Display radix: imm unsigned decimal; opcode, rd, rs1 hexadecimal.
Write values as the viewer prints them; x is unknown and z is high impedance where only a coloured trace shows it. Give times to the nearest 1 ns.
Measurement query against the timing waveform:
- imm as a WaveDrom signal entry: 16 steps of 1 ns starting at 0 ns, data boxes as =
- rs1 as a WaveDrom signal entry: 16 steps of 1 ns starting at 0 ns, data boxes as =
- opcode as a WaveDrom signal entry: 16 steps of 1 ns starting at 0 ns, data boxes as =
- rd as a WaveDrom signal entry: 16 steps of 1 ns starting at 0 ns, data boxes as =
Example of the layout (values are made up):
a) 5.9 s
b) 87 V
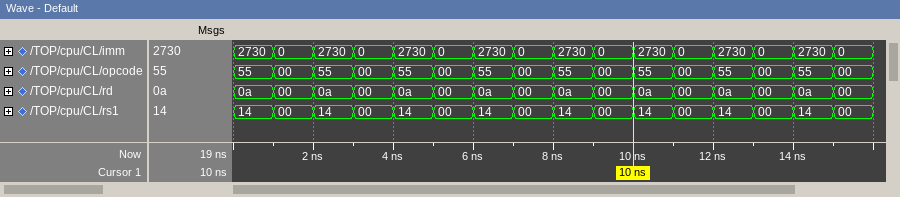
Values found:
a) {name: 'imm', wave: '================', data: '2730 0 2730 0 2730 0 2730 0 2730 0 2730 0 2730 0 2730 0'}
b) {name: 'rs1', wave: '================', data: '14 00 14 00 14 00 14 00 14 00 14 00 14 00 14 00'}
c) {name: 'opcode', wave: '================', data: '55 00 55 00 55 00 55 00 55 00 55 00 55 00 55 00'}
d) {name: 'rd', wave: '================', data: '0a 00 0a 00 0a 00 0a 00 0a 00 0a 00 0a 00 0a 00'}
